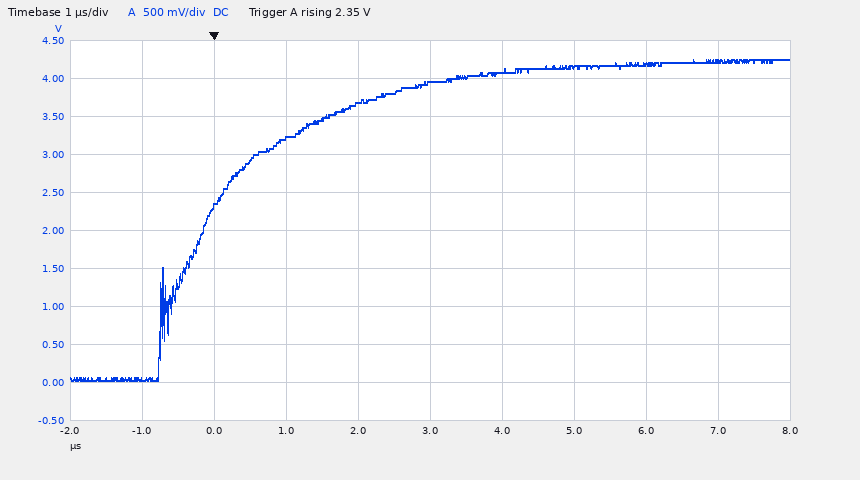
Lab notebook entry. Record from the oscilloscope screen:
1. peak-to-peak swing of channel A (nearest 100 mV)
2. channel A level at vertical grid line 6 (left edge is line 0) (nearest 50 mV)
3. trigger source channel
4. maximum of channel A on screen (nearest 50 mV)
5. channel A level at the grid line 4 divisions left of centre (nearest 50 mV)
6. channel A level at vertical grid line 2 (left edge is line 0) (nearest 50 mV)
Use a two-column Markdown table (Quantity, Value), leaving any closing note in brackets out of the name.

| Quantity | Value |
|---|---|
| peak-to-peak swing of channel A | 4.20 V |
| channel A level at vertical grid line 6 (left edge is line 0) | 4.10 V |
| trigger source channel | channel A |
| maximum of channel A on screen | 4.25 V |
| channel A level at the grid line 4 divisions left of centre | 50 mV |
| channel A level at vertical grid line 2 (left edge is line 0) | 2.30 V |
